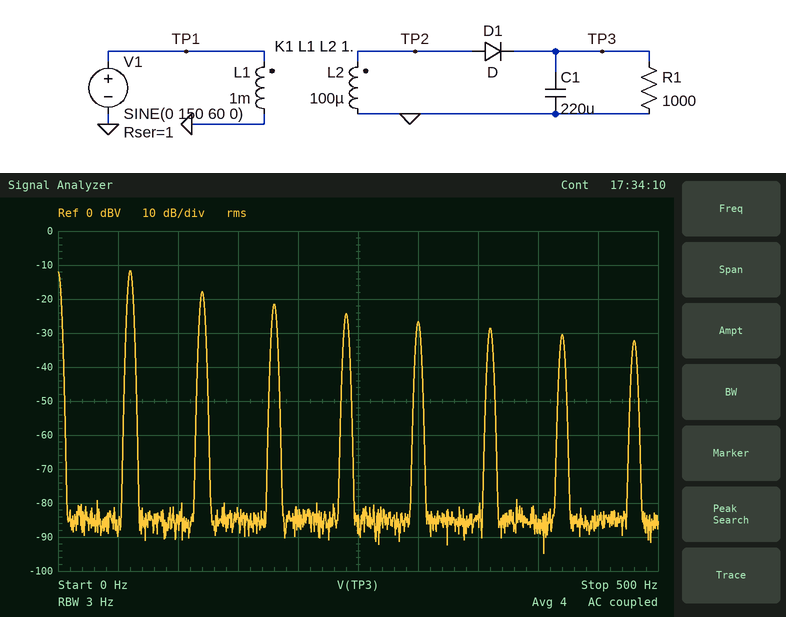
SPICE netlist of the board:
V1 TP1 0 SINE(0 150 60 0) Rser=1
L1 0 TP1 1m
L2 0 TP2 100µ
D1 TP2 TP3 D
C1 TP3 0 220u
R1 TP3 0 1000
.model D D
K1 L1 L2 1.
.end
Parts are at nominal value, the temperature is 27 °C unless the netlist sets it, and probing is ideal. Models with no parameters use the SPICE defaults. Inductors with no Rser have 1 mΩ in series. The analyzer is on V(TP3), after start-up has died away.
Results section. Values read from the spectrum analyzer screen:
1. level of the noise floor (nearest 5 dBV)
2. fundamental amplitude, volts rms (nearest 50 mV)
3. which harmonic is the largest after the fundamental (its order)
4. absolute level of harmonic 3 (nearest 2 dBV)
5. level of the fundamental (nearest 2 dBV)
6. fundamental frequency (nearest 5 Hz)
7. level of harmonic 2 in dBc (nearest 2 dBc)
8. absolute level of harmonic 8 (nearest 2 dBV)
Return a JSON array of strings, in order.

["-85 dBV", "250 mV", "2", "-22 dBV", "-12 dBV", "60 Hz", "-6 dBc", "-32 dBV"]
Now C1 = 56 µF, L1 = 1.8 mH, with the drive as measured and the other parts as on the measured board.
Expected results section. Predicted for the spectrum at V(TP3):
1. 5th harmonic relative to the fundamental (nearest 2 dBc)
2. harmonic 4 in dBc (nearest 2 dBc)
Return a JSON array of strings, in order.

["-18 dBc", "-14 dBc"]
